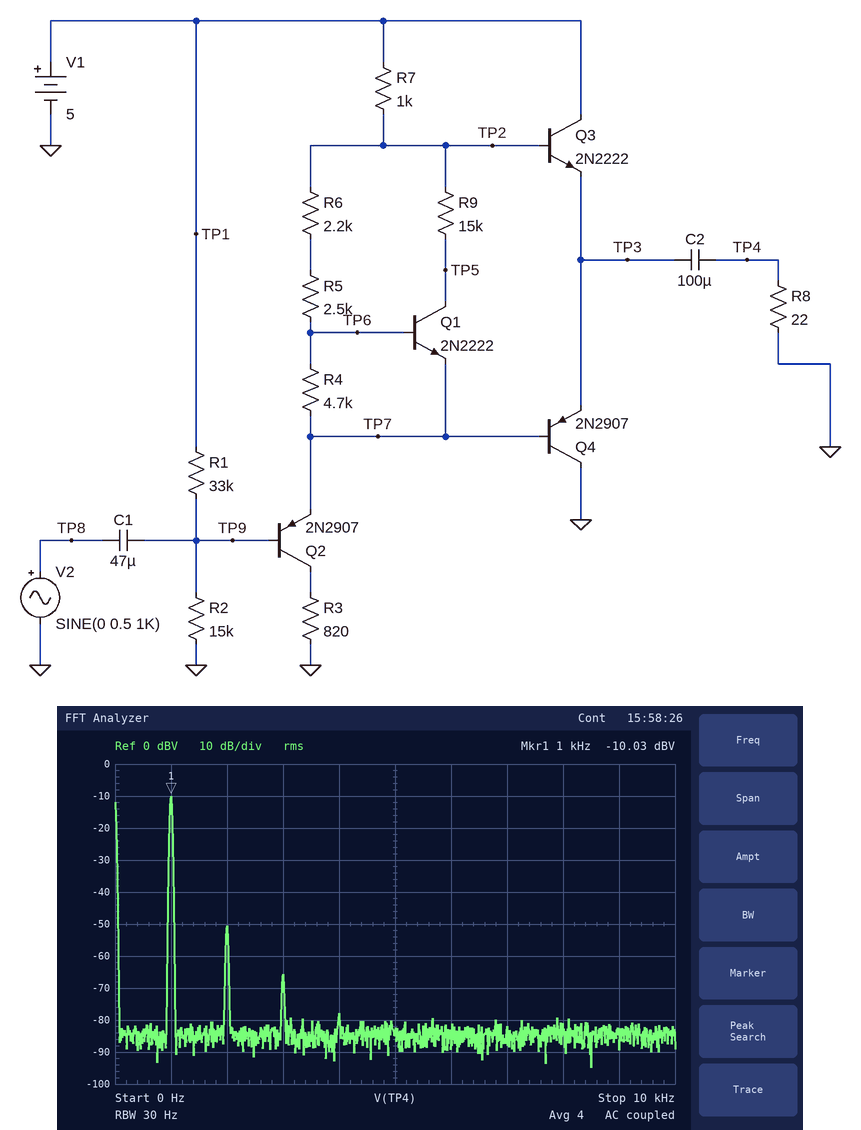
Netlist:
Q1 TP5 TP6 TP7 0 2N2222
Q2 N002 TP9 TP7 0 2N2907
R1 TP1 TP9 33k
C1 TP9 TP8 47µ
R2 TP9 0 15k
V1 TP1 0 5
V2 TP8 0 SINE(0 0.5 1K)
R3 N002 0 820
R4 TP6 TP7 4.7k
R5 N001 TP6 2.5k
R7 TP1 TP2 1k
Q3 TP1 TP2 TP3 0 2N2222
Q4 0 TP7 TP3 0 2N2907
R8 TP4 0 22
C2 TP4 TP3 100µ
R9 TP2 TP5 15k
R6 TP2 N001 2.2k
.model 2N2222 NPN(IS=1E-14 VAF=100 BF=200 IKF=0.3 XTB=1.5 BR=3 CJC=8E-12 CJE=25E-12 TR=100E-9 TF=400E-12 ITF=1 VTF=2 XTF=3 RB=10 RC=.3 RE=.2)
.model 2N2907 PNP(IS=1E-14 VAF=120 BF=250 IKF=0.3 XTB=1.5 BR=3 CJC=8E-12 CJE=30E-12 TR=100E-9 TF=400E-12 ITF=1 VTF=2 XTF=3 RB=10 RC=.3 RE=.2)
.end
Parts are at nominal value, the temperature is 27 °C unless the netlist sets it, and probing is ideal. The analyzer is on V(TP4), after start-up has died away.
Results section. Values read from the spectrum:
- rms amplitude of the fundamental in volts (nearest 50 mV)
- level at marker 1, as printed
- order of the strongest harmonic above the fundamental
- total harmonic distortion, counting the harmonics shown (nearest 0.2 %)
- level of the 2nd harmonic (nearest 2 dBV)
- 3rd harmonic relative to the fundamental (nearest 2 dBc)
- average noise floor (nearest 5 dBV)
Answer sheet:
300 mV
-10.03 dBV
2
1.0 %
-50 dBV
-56 dBc
-85 dBV
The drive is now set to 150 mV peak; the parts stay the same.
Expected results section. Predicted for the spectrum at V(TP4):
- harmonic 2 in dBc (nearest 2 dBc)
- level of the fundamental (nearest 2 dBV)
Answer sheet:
-52 dBc
-20 dBV
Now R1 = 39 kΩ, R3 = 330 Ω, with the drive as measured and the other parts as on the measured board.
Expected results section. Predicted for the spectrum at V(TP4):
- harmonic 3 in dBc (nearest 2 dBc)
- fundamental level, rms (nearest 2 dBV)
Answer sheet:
-60 dBc
-10 dBV
